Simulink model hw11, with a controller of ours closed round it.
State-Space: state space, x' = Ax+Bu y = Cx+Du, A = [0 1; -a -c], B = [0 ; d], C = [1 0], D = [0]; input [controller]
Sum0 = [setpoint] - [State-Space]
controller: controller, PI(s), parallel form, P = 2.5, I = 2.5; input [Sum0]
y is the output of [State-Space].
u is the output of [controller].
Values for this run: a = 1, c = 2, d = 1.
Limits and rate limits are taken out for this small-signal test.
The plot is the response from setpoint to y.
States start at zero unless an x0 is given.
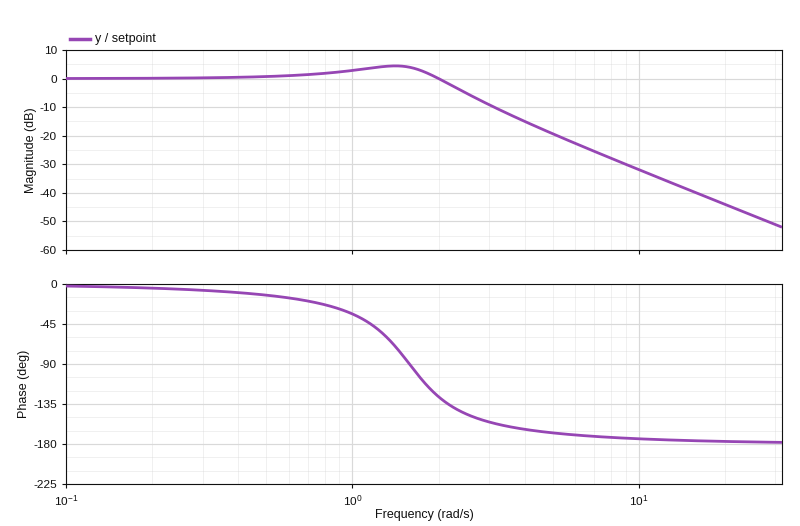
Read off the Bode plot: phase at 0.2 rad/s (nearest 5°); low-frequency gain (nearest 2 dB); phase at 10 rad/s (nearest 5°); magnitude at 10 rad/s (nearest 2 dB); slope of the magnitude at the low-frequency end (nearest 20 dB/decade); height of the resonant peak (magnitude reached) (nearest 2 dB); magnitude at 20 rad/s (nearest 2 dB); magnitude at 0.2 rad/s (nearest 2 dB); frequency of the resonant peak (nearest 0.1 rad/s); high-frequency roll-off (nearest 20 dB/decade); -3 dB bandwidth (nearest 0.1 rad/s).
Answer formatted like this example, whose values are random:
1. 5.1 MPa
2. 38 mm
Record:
1. -5°
2. 0 dB
3. -175°
4. -32 dB
5. 0 dB/decade
6. 4 dB
7. -44 dB
8. 0 dB
9. 1.4 rad/s
10. -40 dB/decade
11. 2.3 rad/s
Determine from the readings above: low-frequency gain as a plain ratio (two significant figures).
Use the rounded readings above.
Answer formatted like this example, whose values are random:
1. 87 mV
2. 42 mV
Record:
1. 1.0
